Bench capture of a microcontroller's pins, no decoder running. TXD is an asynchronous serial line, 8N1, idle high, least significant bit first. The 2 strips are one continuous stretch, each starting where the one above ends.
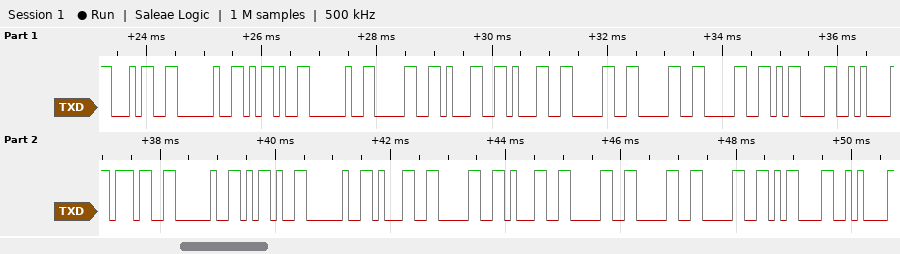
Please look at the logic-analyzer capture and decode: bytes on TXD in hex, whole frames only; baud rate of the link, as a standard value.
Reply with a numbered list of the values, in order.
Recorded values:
1. 0x34 0x20 0x2D 0x20 0x30 0x31 0x31 0x30 0x30 0x30 0x0D 0x0A 0x37 0x20 0x2D 0x20 0x31 0x30 0x31 0x30 0x30 0x30 0x0D 0x0A
2. 9600 baud
